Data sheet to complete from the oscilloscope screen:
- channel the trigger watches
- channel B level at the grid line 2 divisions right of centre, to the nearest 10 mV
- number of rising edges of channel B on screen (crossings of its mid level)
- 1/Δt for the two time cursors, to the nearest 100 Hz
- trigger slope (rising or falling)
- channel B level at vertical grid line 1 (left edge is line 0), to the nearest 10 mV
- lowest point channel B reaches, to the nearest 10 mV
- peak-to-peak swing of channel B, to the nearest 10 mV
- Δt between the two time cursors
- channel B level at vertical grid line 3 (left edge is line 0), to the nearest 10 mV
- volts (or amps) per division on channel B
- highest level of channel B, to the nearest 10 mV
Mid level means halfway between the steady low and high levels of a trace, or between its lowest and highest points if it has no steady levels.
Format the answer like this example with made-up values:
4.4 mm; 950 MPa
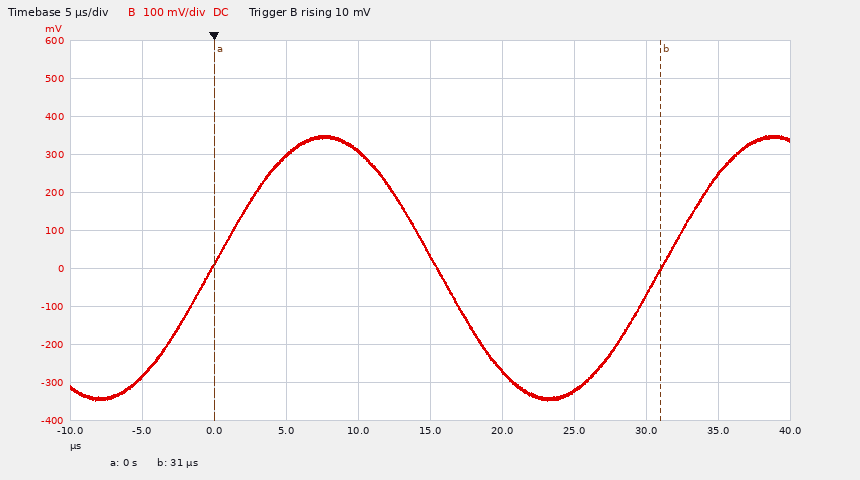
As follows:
channel B; -320 mV; 2; 32.3 kHz; rising; -280 mV; -350 mV; 700 mV; 31.0 µs; 300 mV; 100 mV; 350 mV
